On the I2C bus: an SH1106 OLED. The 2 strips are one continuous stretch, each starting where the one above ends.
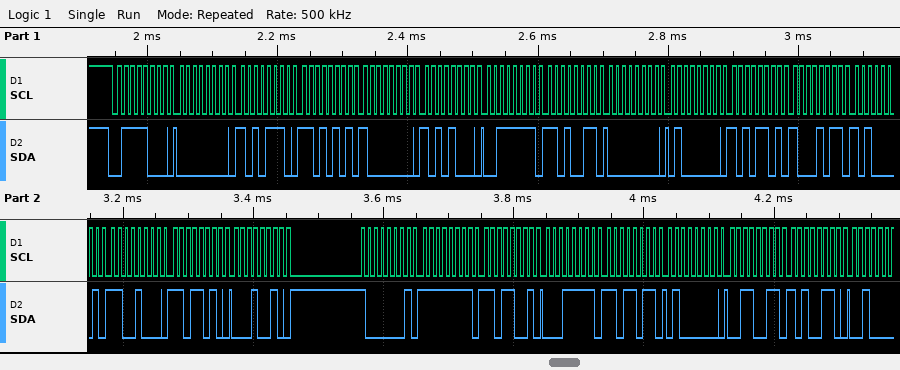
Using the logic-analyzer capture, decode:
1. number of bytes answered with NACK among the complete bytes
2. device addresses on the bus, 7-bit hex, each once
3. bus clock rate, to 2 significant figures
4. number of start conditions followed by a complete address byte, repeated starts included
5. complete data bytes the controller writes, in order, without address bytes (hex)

0
0x3C
100 kHz
1
00 AE D5 80 A8 3F D3 00 40 AD 8B A1 C8 DA 12 81 FF D9 1F DB 40 33 A6
